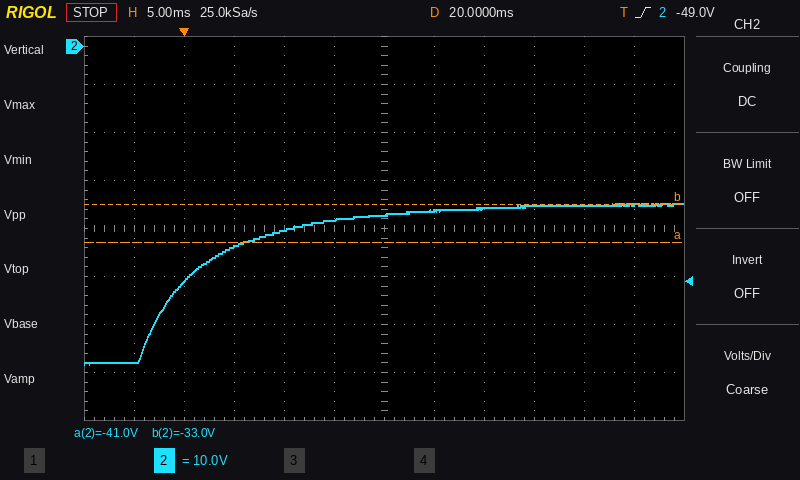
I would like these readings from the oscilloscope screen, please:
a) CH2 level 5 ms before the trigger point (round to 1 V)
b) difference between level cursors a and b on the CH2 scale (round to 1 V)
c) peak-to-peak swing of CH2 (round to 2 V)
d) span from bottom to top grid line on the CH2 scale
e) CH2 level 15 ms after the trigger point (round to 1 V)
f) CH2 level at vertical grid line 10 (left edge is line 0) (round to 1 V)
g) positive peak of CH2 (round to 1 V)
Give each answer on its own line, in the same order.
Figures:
-66 V
8 V
34 V
80 V
-36 V
-33 V
-33 V
